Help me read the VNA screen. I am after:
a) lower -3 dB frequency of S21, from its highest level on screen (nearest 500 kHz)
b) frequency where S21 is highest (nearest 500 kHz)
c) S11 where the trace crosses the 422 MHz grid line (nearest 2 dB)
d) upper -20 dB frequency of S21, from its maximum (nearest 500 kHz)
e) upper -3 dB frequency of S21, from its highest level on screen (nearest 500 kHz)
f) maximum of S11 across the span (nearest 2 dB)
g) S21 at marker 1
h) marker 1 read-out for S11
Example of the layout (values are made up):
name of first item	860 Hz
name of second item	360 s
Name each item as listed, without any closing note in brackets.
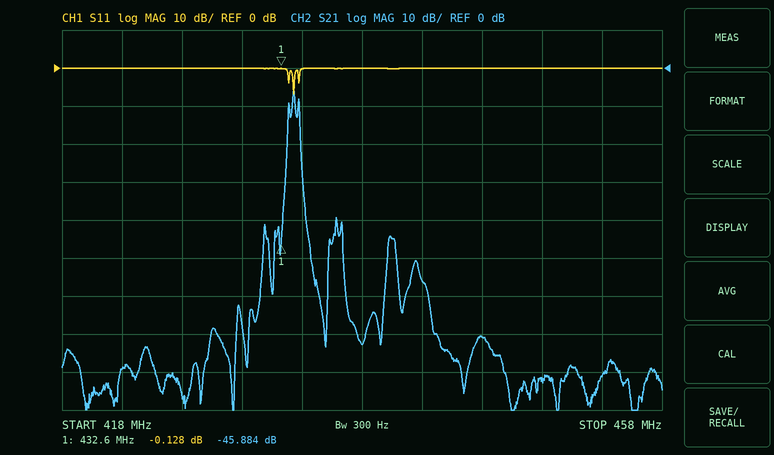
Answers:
lower -3 dB frequency of S21, from its highest level on screen	433.5 MHz
frequency where S21 is highest	433.5 MHz
S11 where the trace crosses the 422 MHz grid line	0 dB
upper -20 dB frequency of S21, from its maximum	434.0 MHz
upper -3 dB frequency of S21, from its highest level on screen	433.5 MHz
maximum of S11 across the span	0 dB
S21 at marker 1	-45.884 dB
marker 1 read-out for S11	-0.128 dB
